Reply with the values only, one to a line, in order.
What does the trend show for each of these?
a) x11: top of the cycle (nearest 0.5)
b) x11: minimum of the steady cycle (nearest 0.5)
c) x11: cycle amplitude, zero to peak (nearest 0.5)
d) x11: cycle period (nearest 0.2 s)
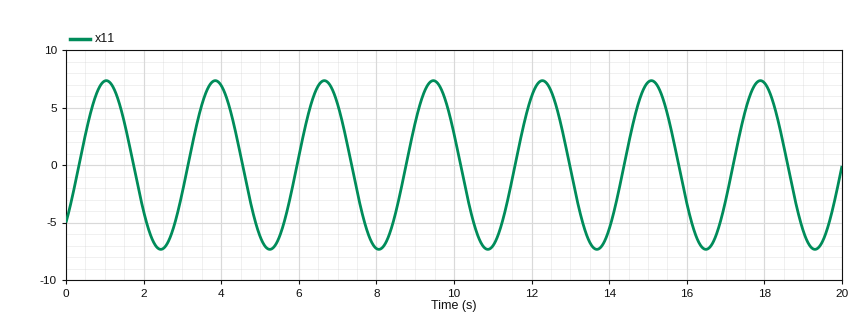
7.5
-7.5
7.5
2.8 s
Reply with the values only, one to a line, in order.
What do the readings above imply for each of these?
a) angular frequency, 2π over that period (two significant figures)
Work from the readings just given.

2.2 rad/s
